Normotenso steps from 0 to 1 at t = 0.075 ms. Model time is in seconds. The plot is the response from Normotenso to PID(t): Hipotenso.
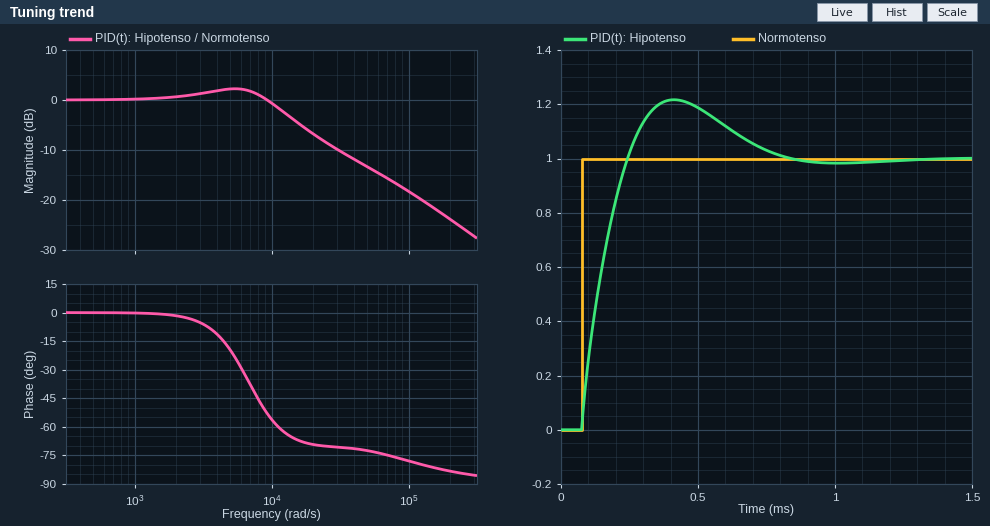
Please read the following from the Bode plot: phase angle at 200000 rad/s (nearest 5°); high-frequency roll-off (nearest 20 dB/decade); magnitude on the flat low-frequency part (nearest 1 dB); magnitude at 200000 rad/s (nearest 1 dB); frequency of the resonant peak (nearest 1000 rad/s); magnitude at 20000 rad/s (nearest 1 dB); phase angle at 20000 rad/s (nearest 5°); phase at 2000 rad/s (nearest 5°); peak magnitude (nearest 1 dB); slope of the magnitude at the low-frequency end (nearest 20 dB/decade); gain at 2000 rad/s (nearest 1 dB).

-85°
-20 dB/decade
0 dB
-24 dB
5000 rad/s
-7 dB
-70°
0°
2 dB
0 dB/decade
1 dB
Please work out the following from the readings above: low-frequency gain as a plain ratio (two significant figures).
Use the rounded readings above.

1.0
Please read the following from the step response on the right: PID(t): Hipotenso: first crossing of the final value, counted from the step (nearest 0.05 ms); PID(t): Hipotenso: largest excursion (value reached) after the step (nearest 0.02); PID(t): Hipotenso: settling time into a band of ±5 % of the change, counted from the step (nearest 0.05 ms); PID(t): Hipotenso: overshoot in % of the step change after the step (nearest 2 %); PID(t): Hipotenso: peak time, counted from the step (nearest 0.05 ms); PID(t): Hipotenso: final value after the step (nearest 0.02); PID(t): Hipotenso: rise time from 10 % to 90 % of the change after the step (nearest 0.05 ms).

0.15 ms
1.22
0.65 ms
22 %
0.35 ms
1.00
0.15 ms
